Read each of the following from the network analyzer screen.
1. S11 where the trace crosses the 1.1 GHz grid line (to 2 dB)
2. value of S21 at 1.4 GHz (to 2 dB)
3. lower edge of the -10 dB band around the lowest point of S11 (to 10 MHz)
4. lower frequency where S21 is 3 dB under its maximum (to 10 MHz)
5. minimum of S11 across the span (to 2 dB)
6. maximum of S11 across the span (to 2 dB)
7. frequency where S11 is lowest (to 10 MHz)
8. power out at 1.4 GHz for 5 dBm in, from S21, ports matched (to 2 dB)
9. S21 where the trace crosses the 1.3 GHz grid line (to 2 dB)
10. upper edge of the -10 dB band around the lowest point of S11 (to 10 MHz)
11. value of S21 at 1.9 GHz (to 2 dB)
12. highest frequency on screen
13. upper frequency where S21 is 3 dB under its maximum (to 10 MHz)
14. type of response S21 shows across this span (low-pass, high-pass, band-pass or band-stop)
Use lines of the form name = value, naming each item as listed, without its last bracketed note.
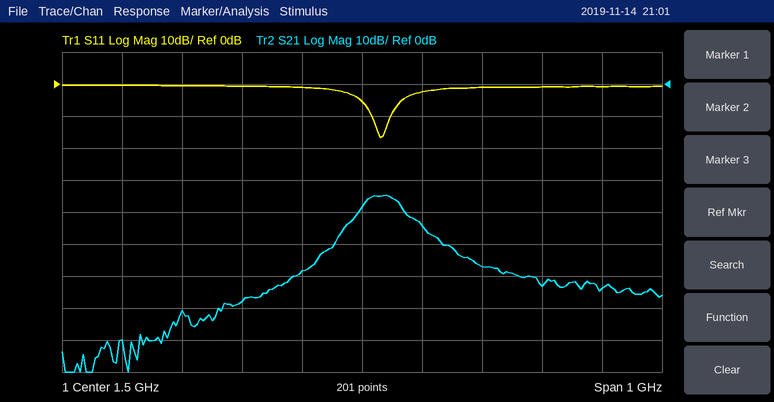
S11 where the trace crosses the 1.1 GHz grid line = 0 dB
value of S21 at 1.4 GHz = -58 dB
lower edge of the -10 dB band around the lowest point of S11 = 1.52 GHz
lower frequency where S21 is 3 dB under its maximum = 1.50 GHz
minimum of S11 across the span = -16 dB
maximum of S11 across the span = 0 dB
frequency where S11 is lowest = 1.53 GHz
power out at 1.4 GHz for 5 dBm in, from S21, ports matched = -54 dBm
S21 where the trace crosses the 1.3 GHz grid line = -68 dB
upper edge of the -10 dB band around the lowest point of S11 = 1.55 GHz
value of S21 at 1.9 GHz = -64 dB
highest frequency on screen = 2 GHz
upper frequency where S21 is 3 dB under its maximum = 1.56 GHz
type of response S21 shows across this span = band-pass
